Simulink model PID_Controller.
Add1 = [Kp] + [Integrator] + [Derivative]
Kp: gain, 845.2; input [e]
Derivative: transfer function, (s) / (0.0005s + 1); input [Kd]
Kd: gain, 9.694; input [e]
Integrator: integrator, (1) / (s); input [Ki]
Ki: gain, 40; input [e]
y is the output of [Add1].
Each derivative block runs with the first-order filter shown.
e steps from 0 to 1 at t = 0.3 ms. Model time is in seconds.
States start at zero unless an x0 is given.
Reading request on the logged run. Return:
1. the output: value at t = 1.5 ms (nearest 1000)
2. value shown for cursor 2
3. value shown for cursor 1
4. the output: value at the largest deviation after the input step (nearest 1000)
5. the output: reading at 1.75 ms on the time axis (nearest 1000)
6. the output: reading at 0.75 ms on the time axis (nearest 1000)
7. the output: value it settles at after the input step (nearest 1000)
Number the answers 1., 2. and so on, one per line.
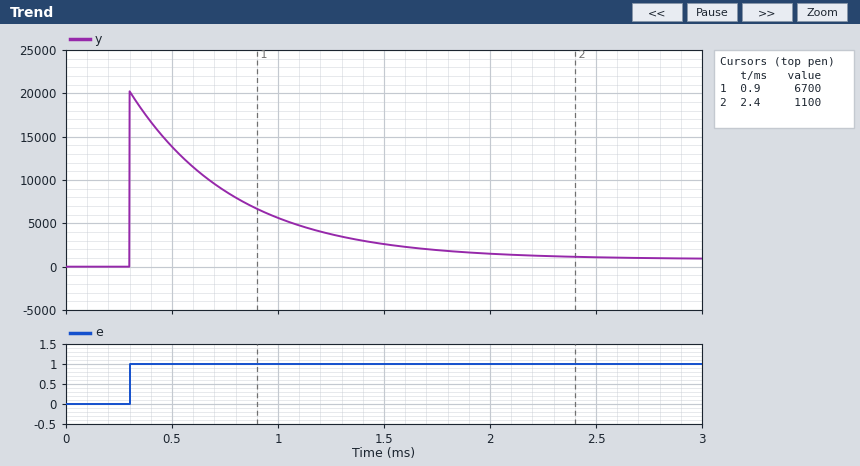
1. 3000
2. 1100
3. 6700
4. 20000
5. 2000
6. 9000
7. 1000
